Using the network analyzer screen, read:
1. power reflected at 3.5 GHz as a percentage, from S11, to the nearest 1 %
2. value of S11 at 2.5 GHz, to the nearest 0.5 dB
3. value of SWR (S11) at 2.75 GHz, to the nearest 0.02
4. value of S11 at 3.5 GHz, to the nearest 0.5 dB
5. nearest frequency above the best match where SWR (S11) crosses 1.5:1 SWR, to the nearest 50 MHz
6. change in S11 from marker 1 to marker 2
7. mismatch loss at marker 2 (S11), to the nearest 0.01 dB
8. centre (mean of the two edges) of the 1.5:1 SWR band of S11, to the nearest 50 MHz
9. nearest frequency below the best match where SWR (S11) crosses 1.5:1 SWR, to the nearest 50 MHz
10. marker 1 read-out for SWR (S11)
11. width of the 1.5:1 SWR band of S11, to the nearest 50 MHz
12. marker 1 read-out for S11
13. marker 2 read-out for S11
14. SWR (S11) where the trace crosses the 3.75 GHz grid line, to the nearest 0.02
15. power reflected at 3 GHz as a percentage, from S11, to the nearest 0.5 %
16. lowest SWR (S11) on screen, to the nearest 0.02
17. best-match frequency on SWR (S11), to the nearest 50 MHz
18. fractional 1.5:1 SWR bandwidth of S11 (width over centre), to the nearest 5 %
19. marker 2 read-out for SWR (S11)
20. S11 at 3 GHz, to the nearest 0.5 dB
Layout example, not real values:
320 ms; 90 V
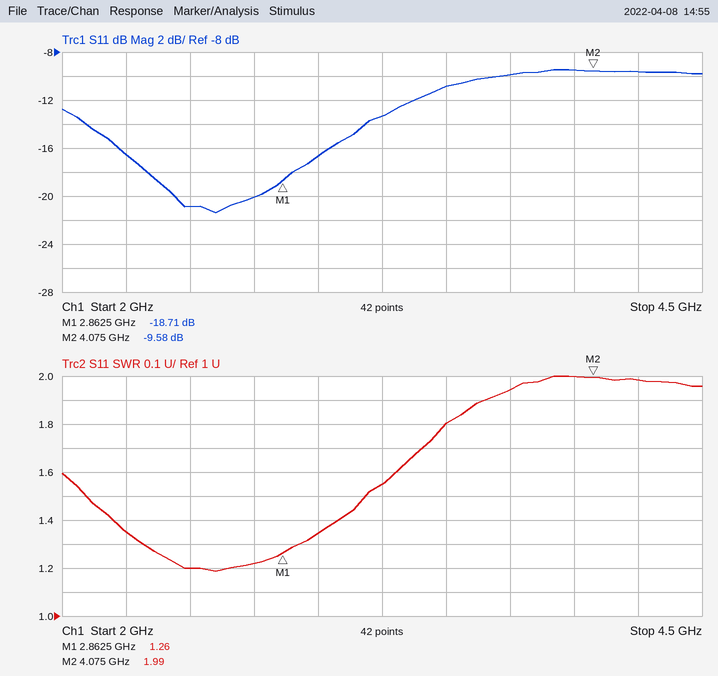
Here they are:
8 %; -21.0 dB; 1.22; -11.0 dB; 3.20 GHz; 9.13 dB; 0.51 dB; 2.65 GHz; 2.10 GHz; 1.26; 1.10 GHz; -18.71 dB; -9.58 dB; 1.94; 2.0 %; 1.18; 2.60 GHz; 40 %; 1.99; -16.5 dB
